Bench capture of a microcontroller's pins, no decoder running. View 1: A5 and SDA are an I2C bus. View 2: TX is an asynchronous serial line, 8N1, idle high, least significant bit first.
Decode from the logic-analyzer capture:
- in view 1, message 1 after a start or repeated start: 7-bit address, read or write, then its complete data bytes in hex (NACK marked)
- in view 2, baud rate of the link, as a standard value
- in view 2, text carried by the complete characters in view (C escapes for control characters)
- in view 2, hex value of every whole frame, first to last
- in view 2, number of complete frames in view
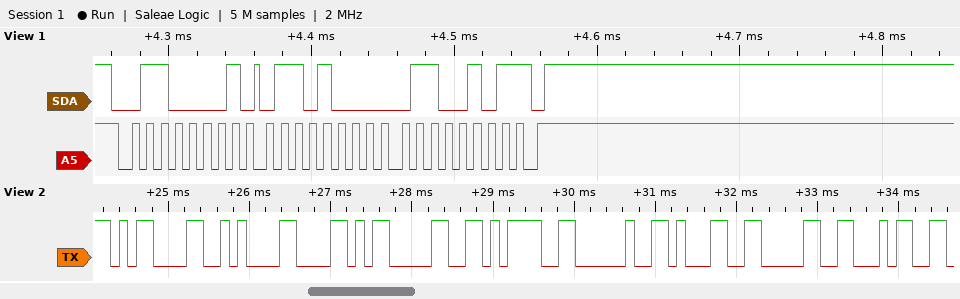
0x30 read: 68 65 NACK
9600 baud
"\r\nX0= 104"
0D 0A 58 30 3D 20 31 30 34
9
